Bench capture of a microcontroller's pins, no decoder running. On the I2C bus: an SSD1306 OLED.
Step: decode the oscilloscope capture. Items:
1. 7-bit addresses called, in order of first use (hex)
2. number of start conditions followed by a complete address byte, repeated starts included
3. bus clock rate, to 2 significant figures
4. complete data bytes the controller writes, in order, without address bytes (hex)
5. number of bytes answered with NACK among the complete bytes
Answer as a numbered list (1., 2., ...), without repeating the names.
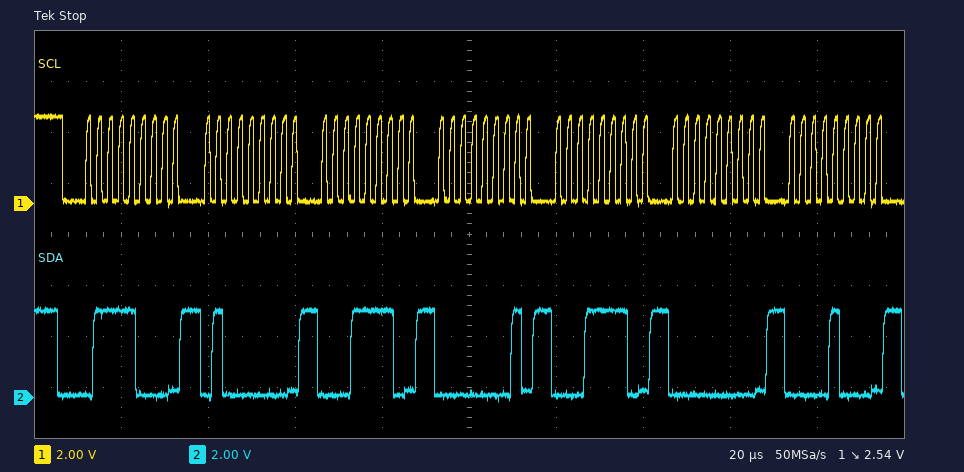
1. 0x3C
2. 1
3. 400 kHz
4. 40 1E 01 1E 00 08
5. 0
